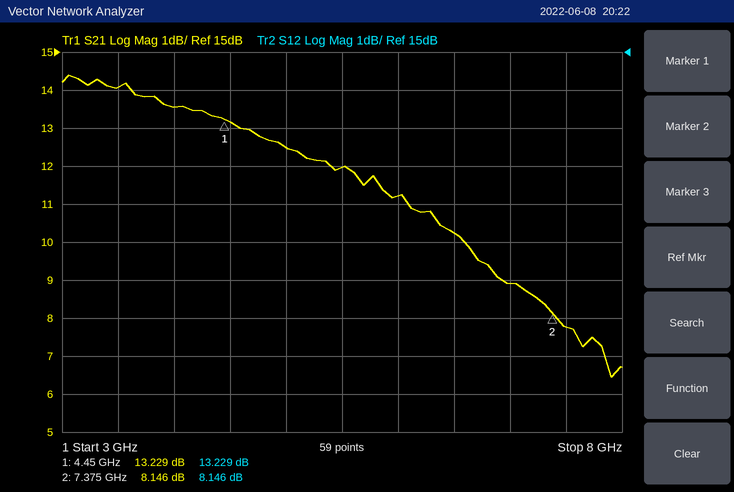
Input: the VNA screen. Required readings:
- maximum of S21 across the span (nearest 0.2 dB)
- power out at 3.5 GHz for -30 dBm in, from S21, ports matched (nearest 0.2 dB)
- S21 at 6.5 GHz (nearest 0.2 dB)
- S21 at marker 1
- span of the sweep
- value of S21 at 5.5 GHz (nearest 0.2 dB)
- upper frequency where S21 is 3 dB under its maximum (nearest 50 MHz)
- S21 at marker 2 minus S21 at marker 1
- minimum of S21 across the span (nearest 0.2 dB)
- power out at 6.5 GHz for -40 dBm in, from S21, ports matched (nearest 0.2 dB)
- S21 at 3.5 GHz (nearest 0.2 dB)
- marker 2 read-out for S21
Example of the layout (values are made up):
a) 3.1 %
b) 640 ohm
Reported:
a) 14.4 dB
b) -16.0 dBm
c) 10.2 dB
d) 13.229 dB
e) 5 GHz
f) 12.0 dB
g) 5.85 GHz
h) -5.083 dB
i) 6.4 dB
j) -29.8 dBm
k) 14.0 dB
l) 8.146 dB
